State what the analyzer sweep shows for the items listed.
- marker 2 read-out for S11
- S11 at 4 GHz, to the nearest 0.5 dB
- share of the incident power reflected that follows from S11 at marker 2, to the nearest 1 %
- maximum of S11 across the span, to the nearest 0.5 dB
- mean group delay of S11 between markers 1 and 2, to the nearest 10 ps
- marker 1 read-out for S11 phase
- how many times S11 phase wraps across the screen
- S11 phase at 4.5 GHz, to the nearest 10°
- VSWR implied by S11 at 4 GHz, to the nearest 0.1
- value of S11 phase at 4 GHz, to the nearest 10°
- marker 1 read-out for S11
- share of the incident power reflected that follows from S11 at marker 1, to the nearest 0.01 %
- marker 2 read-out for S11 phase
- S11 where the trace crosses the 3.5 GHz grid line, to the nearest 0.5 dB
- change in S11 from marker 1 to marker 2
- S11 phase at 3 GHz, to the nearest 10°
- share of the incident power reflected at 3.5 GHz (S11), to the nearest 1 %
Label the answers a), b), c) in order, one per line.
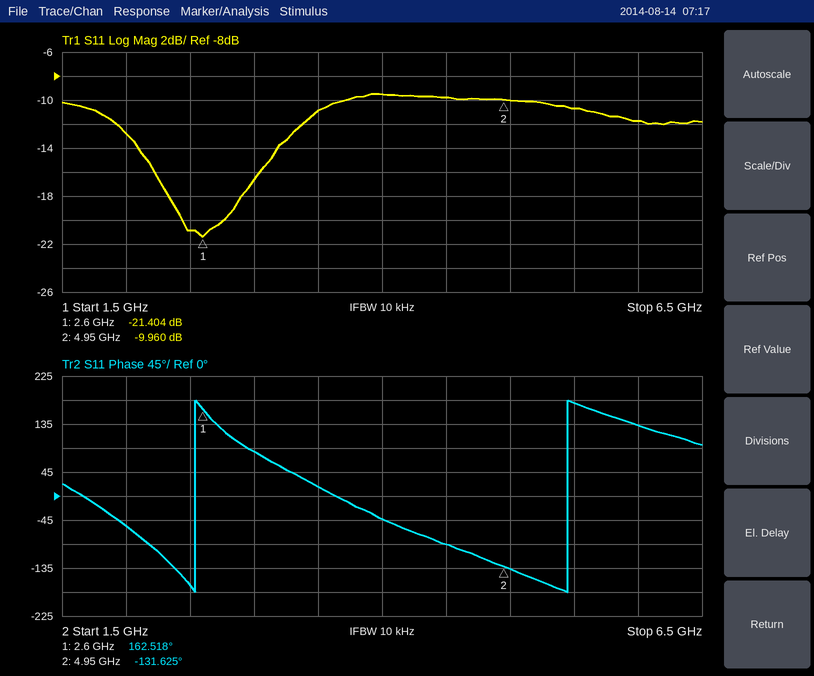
a) -9.960 dB
b) -9.5 dB
c) 10 %
d) -9.5 dB
e) 350 ps
f) 162.518°
g) 2
h) -90°
i) 2.0
j) -40°
k) -21.404 dB
l) 0.72 %
m) -131.625°
n) -11.0 dB
o) 11.444 dB
p) 80°
q) 8 %
